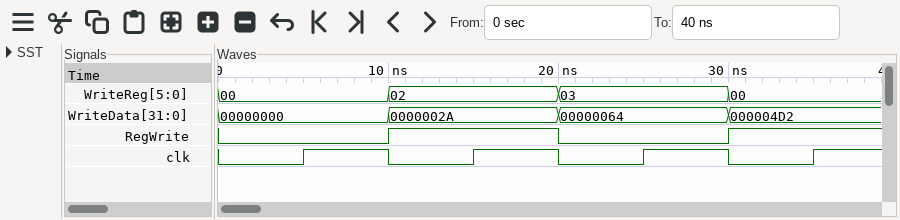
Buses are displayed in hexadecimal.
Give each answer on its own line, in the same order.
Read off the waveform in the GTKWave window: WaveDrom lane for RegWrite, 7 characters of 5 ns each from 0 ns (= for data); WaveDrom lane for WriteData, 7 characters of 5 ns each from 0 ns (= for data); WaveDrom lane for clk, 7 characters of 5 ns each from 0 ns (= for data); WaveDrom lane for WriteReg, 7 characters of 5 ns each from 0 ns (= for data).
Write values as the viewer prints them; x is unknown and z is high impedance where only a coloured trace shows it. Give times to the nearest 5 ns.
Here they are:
{name: 'RegWrite', wave: '0.1.0.1'}
{name: 'WriteData', wave: '=.=.=.=', data: '00000000 0000002A 00000064 000004D2'}
{name: 'clk', wave: '0101010'}
{name: 'WriteReg', wave: '=.=.=.=', data: '00 02 03 00'}
